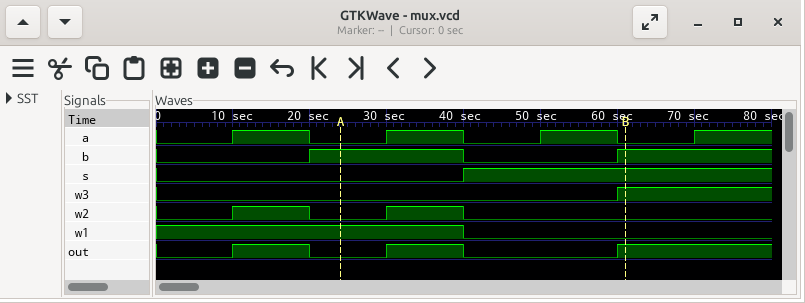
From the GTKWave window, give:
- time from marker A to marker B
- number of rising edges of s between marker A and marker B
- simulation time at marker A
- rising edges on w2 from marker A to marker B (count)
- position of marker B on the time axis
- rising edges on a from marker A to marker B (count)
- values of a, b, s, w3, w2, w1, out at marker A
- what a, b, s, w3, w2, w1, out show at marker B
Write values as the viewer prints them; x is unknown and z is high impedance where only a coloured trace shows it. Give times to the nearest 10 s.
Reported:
40 s
1
20 s
1
60 s
2
a=0, b=1, s=0, w3=0, w2=0, w1=1, out=0
a=0, b=1, s=1, w3=1, w2=0, w1=0, out=1
